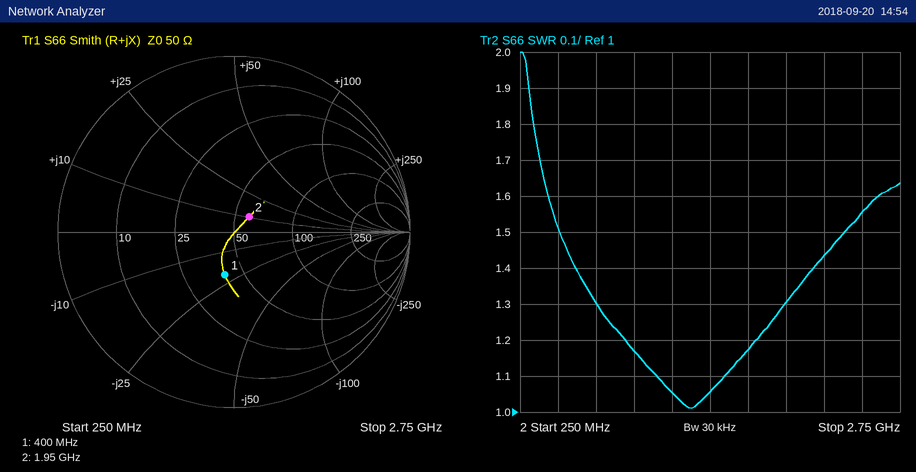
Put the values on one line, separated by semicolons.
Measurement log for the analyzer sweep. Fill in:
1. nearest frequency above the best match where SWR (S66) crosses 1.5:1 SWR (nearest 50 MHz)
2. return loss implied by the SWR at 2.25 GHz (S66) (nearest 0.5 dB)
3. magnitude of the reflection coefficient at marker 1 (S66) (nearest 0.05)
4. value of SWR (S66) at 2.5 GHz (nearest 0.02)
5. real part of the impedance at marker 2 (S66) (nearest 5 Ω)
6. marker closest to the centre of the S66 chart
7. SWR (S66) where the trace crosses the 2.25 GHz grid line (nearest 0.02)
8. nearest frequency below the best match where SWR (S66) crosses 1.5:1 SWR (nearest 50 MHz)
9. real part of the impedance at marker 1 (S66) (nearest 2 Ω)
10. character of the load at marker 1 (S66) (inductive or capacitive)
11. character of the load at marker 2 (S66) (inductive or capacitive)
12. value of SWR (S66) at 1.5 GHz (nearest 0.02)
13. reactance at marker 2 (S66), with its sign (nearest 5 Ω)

2.40 GHz; 15.0 dB; 0.25; 1.56; 60 Ω; marker 2; 1.44; 500 MHz; 40 Ω; capacitive; inductive; 1.06; +10 Ω
